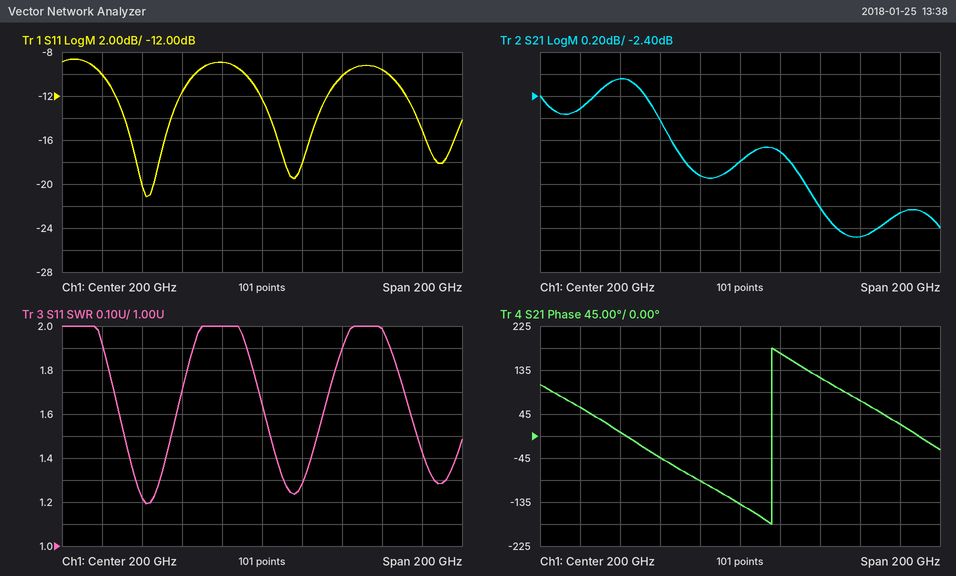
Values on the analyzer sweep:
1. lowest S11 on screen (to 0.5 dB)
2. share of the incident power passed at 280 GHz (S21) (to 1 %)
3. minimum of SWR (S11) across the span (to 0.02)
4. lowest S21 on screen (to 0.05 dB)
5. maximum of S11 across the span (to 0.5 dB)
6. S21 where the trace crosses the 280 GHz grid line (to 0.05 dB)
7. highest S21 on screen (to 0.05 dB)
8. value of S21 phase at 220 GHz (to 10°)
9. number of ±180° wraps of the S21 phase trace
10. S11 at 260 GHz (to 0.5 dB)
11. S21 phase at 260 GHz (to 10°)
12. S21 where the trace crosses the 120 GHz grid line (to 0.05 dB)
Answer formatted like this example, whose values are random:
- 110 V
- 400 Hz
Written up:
- -21.0 dB
- 45 %
- 1.20
- -3.70 dB
- -8.5 dB
- -3.45 dB
- -2.25 dB
- 170°
- 1
- -9.5 dB
- 70°
- -2.50 dB
